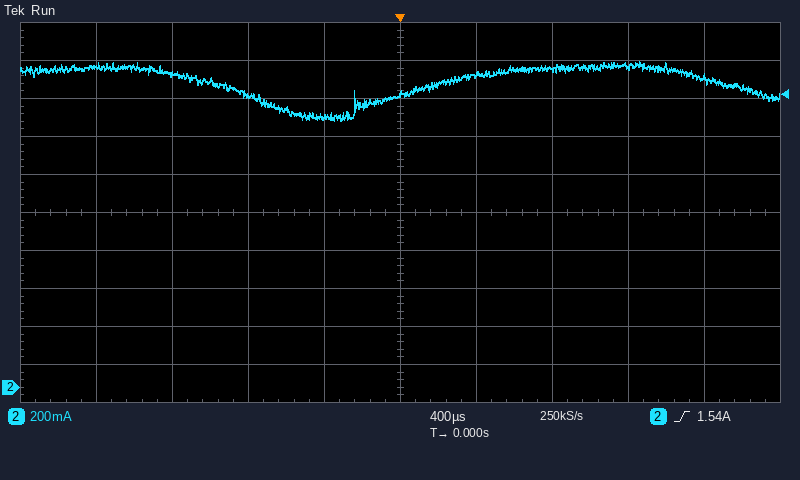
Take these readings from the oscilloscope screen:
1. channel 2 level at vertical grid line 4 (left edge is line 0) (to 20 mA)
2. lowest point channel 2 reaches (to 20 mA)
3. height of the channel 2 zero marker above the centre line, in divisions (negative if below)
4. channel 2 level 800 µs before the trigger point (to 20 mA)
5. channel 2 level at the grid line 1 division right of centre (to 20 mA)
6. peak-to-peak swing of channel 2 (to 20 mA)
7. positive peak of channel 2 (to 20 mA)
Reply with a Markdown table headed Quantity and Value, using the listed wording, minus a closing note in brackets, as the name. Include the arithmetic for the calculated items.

| Quantity | Value |
|---|---|
| channel 2 level at vertical grid line 4 (left edge is line 0) | 1.42 A |
| lowest point channel 2 reaches | 1.40 A |
| height of the channel 2 zero marker above the centre line, in divisions | -4.6 div |
| channel 2 level 800 µs before the trigger point | 1.54 A |
| channel 2 level at the grid line 1 division right of centre | 1.64 A |
| peak-to-peak swing of channel 2 | 1.72 A − (1.40 A) = 320 mA |
| positive peak of channel 2 | 1.72 A |
